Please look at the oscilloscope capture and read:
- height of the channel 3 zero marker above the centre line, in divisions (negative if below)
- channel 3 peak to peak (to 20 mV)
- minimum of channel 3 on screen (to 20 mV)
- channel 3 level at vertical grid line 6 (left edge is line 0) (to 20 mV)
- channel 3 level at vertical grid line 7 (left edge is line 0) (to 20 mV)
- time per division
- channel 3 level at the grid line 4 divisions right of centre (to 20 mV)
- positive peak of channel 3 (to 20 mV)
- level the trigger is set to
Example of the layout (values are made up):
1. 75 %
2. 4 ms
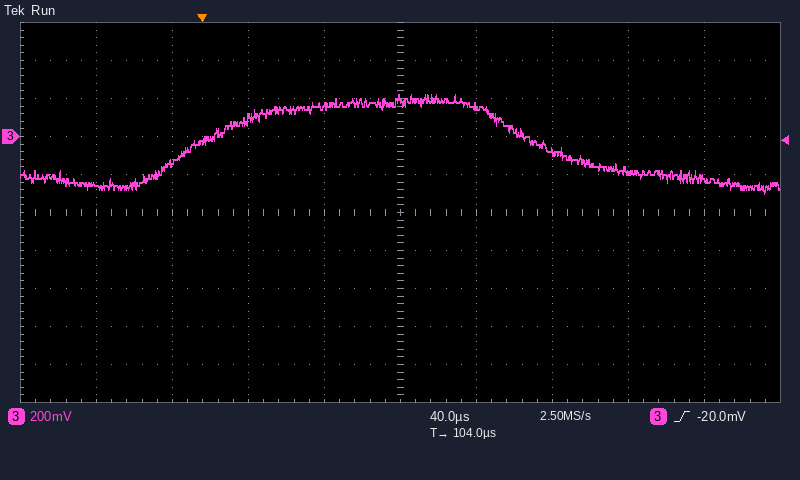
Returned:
1. +2.0 div
2. 520 mV
3. -300 mV
4. 160 mV
5. -80 mV
6. 40 µs
7. -220 mV
8. 220 mV
9. -20.0 mV
